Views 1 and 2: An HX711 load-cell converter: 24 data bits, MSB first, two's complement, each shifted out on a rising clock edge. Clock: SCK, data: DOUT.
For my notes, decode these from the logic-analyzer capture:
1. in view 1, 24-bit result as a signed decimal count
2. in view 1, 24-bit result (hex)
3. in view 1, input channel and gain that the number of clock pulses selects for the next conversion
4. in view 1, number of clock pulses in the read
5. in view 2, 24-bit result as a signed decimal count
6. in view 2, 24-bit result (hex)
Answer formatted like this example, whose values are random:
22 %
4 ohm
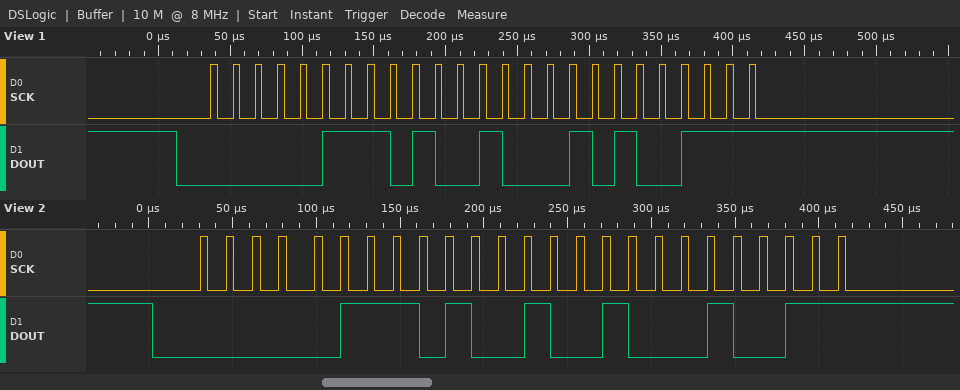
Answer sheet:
477351
0x0748A7
channel A, gain 128
25
477459
0x074913
